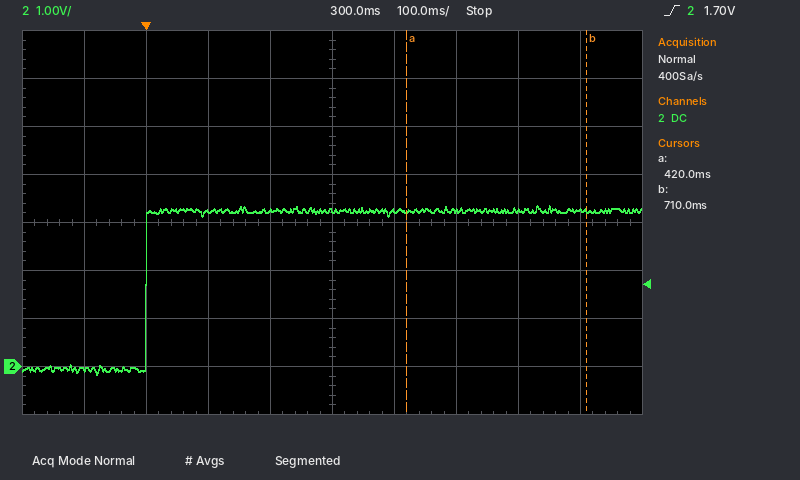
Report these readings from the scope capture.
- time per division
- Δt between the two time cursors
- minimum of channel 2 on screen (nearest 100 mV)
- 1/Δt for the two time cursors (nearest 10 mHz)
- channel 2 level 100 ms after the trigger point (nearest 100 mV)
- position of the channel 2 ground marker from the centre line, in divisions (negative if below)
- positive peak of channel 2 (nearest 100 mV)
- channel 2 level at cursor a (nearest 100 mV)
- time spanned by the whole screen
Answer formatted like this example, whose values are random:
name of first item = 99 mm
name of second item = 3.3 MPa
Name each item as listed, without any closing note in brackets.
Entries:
time per division = 100 ms
Δt between the two time cursors = 290 ms
minimum of channel 2 on screen = -200 mV
1/Δt for the two time cursors = 3.45 Hz
channel 2 level 100 ms after the trigger point = 3.2 V
position of the channel 2 ground marker from the centre line, in divisions = -3.0 div
positive peak of channel 2 = 3.4 V
channel 2 level at cursor a = 3.2 V
time spanned by the whole screen = 1 s
